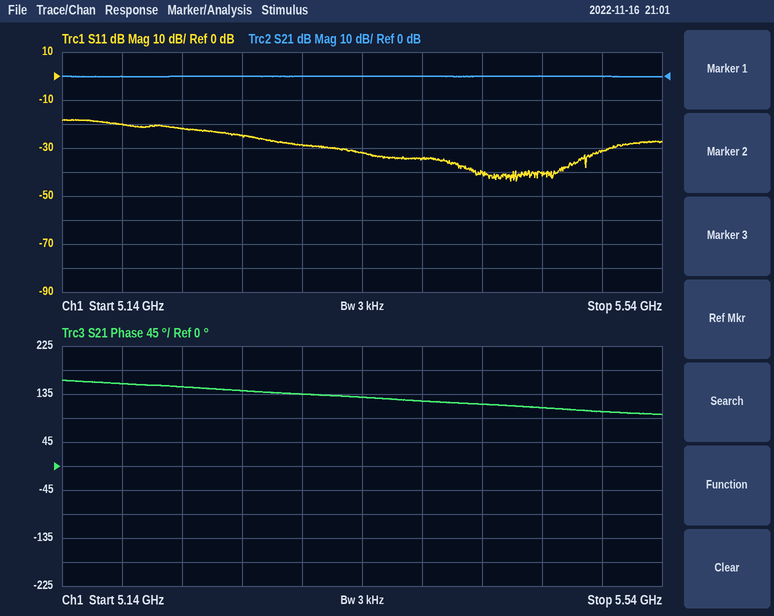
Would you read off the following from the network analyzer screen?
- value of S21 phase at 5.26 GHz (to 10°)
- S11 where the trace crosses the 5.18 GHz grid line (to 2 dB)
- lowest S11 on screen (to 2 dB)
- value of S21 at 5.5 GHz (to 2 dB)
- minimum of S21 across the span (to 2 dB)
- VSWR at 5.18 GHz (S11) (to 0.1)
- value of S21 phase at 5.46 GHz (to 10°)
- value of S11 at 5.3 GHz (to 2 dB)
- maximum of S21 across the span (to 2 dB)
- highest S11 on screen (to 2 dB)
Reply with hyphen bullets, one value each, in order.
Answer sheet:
- 140°
- -20 dB
- -44 dB
- 0 dB
- 0 dB
- 1.2
- 110°
- -28 dB
- 0 dB
- -18 dB
